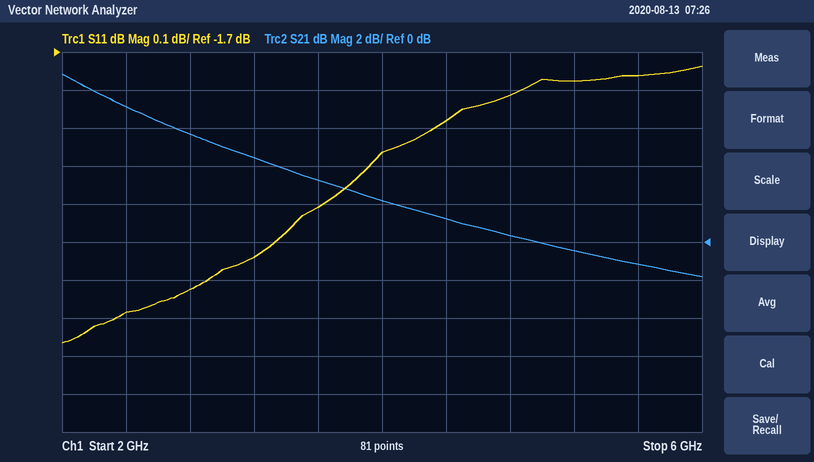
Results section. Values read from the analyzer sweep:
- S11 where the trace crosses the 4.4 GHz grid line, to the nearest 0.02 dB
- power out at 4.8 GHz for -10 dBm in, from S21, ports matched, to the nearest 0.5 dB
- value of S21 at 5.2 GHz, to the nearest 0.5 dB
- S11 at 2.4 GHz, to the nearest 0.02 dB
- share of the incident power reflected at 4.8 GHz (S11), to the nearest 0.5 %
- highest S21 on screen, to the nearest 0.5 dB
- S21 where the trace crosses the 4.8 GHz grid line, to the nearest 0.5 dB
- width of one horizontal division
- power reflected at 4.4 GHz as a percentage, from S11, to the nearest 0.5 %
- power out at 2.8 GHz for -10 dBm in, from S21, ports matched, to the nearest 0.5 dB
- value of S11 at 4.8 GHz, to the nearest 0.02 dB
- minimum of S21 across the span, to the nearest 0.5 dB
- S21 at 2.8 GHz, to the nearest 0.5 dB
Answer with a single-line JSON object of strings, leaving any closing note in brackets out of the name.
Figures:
{"S11 where the trace crosses the 4.4 GHz grid line, to the nearest 0.02 dB": "-1.88 dB", "power out at 4.8 GHz for -10 dBm in, from S21, ports matched, to the nearest 0.5 dB": "-9.5 dBm", "value of S21 at 5.2 GHz, to the nearest 0.5 dB": "-0.5 dB", "S11 at 2.4 GHz, to the nearest 0.02 dB": "-2.38 dB", "share of the incident power reflected at 4.8 GHz (S11), to the nearest 0.5 %": "66.0 %", "highest S21 on screen, to the nearest 0.5 dB": "9.0 dB", "S21 where the trace crosses the 4.8 GHz grid line, to the nearest 0.5 dB": "0.5 dB", "width of one horizontal division": "400 MHz", "power reflected at 4.4 GHz as a percentage, from S11, to the nearest 0.5 %": "65.0 %", "power out at 2.8 GHz for -10 dBm in, from S21, ports matched, to the nearest 0.5 dB": "-4.5 dBm", "value of S11 at 4.8 GHz, to the nearest 0.02 dB": "-1.82 dB", "minimum of S21 across the span, to the nearest 0.5 dB": "-2.0 dB", "S21 at 2.8 GHz, to the nearest 0.5 dB": "5.5 dB"}
